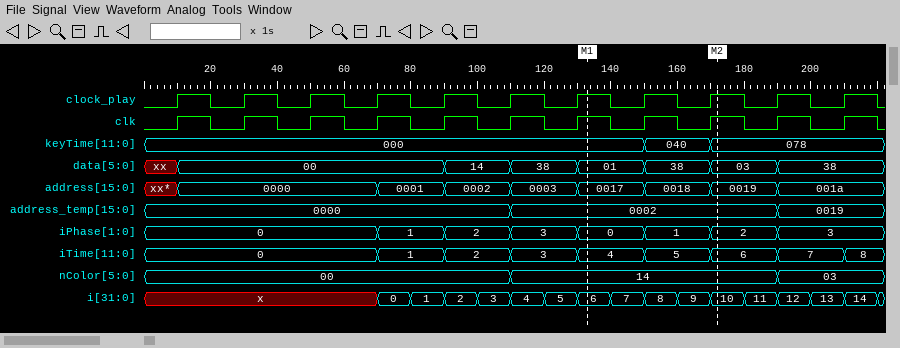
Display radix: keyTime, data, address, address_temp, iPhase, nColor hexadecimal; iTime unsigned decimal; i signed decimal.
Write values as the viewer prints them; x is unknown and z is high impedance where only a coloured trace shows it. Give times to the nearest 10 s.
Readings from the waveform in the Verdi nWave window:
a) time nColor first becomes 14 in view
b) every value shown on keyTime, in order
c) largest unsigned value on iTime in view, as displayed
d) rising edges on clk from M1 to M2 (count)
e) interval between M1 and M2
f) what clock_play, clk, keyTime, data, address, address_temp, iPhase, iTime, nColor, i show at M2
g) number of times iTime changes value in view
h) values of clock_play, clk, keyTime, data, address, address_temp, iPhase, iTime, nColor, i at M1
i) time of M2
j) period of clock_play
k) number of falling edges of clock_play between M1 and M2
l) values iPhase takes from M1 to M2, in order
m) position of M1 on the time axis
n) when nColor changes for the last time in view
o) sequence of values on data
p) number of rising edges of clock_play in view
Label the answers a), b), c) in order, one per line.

a) 110 s
b) 000, 040, 078
c) 8
d) 2
e) 40 s
f) clock_play=1, clk=1, keyTime=078, data=03, address=0019, address_temp=0002, iPhase=2, iTime=6, nColor=14, i=10
g) 8
h) clock_play=1, clk=1, keyTime=000, data=01, address=0017, address_temp=0002, iPhase=0, iTime=4, nColor=14, i=6
i) 170 s
j) 20 s
k) 2
l) 0, 1, 2
m) 130 s
n) 190 s
o) xx, 00, 14, 38, 01, 38, 03, 38
p) 11
